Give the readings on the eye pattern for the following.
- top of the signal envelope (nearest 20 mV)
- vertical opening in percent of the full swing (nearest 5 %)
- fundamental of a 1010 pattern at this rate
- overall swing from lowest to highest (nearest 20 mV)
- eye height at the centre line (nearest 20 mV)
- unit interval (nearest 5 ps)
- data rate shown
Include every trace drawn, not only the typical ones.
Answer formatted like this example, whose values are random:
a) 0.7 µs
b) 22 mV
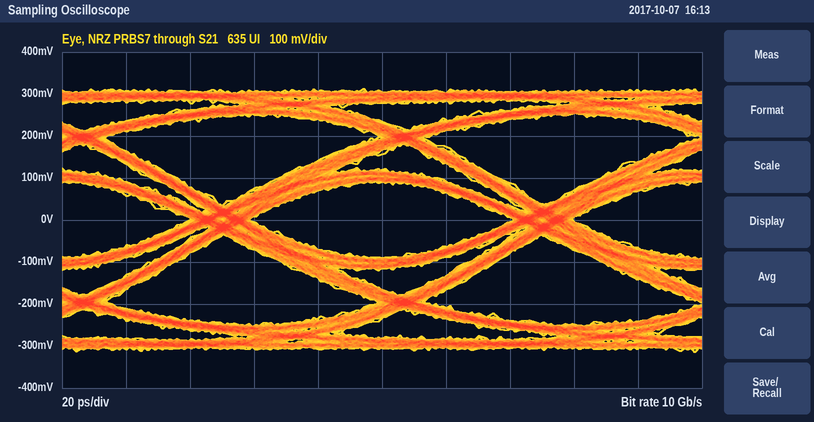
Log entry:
a) 320 mV
b) 30 %
c) 5 GHz
d) 620 mV
e) 180 mV
f) 100 ps
g) 10 Gb/s
